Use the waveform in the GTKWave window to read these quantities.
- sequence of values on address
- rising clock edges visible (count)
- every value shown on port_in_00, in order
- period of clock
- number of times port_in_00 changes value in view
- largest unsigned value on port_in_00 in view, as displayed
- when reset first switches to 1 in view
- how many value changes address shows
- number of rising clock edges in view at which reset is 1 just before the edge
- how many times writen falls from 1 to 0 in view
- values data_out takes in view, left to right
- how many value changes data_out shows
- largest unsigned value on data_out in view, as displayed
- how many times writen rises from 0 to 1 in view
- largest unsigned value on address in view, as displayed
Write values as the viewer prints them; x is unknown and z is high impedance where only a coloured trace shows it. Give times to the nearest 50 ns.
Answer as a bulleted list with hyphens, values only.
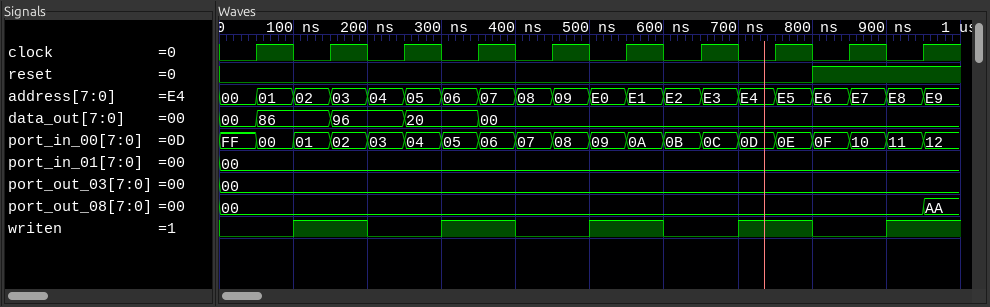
- 00, 01, 02, 03, 04, 05, 06, 07, 08, 09, E0, E1, E2, E3, E4, E5, E6, E7, E8, E9
- 10
- FF, 00, 01, 02, 03, 04, 05, 06, 07, 08, 09, 0A, 0B, 0C, 0D, 0E, 0F, 10, 11, 12
- 100 ns
- 19
- FF
- 800 ns
- 19
- 2
- 4
- 00, 86, 96, 20, 00
- 4
- 96
- 5
- E9
